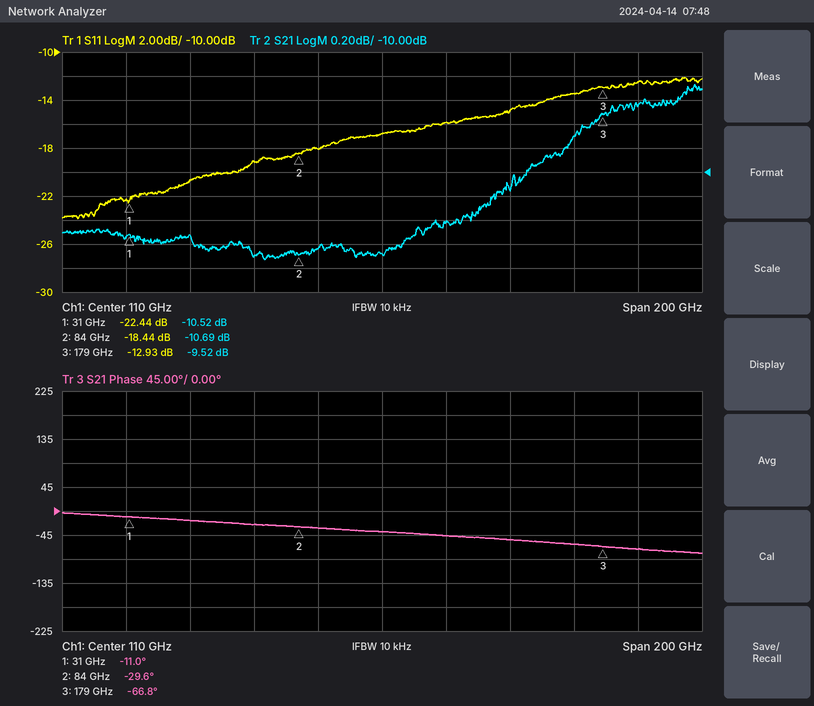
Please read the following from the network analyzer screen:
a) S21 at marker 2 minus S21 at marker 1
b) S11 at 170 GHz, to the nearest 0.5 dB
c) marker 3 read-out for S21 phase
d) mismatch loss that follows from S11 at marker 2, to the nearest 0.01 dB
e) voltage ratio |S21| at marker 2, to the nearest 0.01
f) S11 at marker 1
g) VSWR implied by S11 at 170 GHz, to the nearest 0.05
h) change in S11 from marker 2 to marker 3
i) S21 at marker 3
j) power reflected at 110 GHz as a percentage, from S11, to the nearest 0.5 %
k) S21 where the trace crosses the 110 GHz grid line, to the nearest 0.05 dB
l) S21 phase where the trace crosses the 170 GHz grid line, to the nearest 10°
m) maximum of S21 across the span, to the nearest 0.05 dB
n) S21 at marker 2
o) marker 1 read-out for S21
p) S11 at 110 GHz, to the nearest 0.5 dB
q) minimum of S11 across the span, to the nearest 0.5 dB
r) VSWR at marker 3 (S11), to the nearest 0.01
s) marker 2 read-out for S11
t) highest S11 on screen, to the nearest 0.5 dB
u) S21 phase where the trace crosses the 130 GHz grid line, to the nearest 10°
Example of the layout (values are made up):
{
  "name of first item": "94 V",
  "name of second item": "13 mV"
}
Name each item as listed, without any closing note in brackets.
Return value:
{
  "S21 at marker 2 minus S21 at marker 1": "-0.17 dB",
  "S11 at 170 GHz, to the nearest 0.5 dB": "-13.5 dB",
  "marker 3 read-out for S21 phase": "-66.8°",
  "mismatch loss that follows from S11 at marker 2, to the nearest 0.01 dB": "0.06 dB",
  "voltage ratio |S21| at marker 2, to the nearest 0.01": "0.29",
  "S11 at marker 1": "-22.44 dB",
  "VSWR implied by S11 at 170 GHz, to the nearest 0.05": "1.55",
  "change in S11 from marker 2 to marker 3": "5.51 dB",
  "S21 at marker 3": "-9.52 dB",
  "power reflected at 110 GHz as a percentage, from S11, to the nearest 0.5 %": "2.0 %",
  "S21 where the trace crosses the 110 GHz grid line, to the nearest 0.05 dB": "-10.70 dB",
  "S21 phase where the trace crosses the 170 GHz grid line, to the nearest 10°": "-60°",
  "maximum of S21 across the span, to the nearest 0.05 dB": "-9.25 dB",
  "S21 at marker 2": "-10.69 dB",
  "marker 1 read-out for S21": "-10.52 dB",
  "S11 at 110 GHz, to the nearest 0.5 dB": "-17.0 dB",
  "minimum of S11 across the span, to the nearest 0.5 dB": "-24.0 dB",
  "VSWR at marker 3 (S11), to the nearest 0.01": "1.58",
  "marker 2 read-out for S11": "-18.44 dB",
  "highest S11 on screen, to the nearest 0.5 dB": "-12.0 dB",
  "S21 phase where the trace crosses the 130 GHz grid line, to the nearest 10°": "-50°"
}
